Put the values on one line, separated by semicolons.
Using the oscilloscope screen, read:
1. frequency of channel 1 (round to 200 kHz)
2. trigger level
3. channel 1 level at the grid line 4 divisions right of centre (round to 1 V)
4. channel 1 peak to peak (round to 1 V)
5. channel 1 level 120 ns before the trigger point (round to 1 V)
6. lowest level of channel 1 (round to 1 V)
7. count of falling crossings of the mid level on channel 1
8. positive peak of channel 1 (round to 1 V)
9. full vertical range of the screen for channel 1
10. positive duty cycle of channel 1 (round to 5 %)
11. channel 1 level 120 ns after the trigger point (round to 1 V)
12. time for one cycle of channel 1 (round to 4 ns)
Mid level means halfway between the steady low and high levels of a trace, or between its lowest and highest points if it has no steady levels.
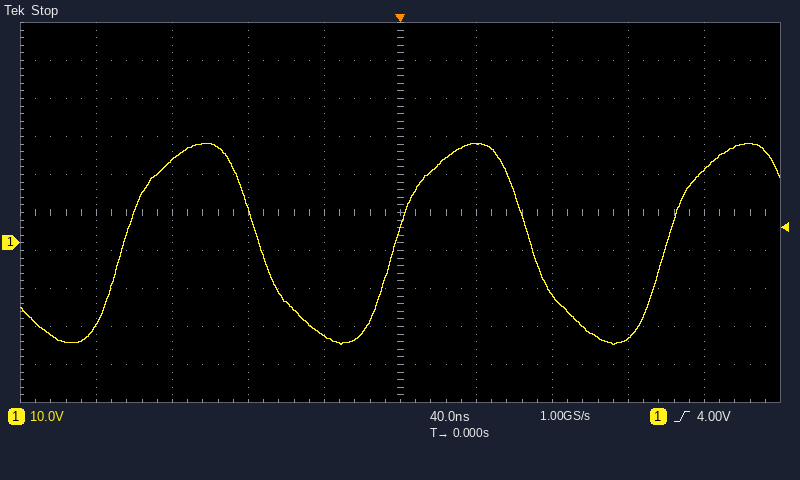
7.0 MHz; 4.00 V; 19 V; 53 V; 22 V; -27 V; 2; 26 V; 100 V; 50 %; -25 V; 144 ns
